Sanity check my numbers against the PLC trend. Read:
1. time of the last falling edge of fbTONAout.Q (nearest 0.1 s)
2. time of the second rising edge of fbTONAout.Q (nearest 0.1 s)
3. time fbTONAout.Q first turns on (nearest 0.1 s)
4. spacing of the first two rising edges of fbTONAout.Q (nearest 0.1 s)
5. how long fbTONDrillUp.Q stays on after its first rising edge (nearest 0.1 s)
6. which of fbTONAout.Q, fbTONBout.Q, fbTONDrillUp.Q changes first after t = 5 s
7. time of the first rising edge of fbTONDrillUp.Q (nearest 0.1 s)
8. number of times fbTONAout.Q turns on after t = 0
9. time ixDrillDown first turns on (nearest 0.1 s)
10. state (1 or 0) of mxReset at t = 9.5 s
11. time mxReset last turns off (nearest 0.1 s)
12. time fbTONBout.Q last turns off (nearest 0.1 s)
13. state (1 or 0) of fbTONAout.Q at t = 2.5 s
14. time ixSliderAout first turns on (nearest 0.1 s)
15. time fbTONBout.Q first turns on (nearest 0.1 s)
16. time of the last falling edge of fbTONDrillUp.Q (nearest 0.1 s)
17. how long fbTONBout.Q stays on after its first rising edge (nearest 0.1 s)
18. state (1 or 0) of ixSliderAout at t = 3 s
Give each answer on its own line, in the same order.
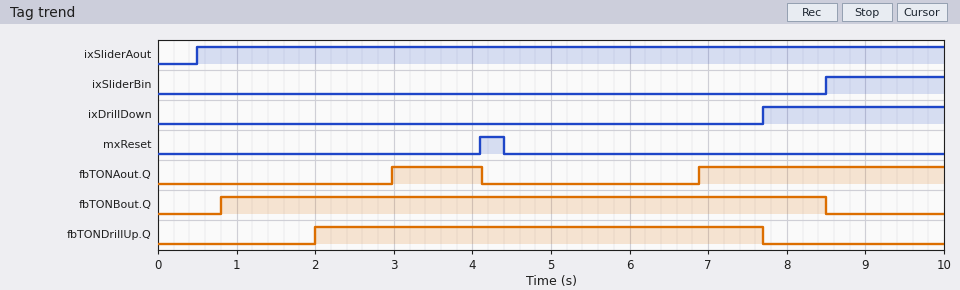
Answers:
4.1 s
6.9 s
3.0 s
3.9 s
5.7 s
fbTONAout.Q
2.0 s
2
7.7 s
0
4.4 s
8.5 s
0
0.5 s
0.8 s
7.7 s
7.7 s
1
